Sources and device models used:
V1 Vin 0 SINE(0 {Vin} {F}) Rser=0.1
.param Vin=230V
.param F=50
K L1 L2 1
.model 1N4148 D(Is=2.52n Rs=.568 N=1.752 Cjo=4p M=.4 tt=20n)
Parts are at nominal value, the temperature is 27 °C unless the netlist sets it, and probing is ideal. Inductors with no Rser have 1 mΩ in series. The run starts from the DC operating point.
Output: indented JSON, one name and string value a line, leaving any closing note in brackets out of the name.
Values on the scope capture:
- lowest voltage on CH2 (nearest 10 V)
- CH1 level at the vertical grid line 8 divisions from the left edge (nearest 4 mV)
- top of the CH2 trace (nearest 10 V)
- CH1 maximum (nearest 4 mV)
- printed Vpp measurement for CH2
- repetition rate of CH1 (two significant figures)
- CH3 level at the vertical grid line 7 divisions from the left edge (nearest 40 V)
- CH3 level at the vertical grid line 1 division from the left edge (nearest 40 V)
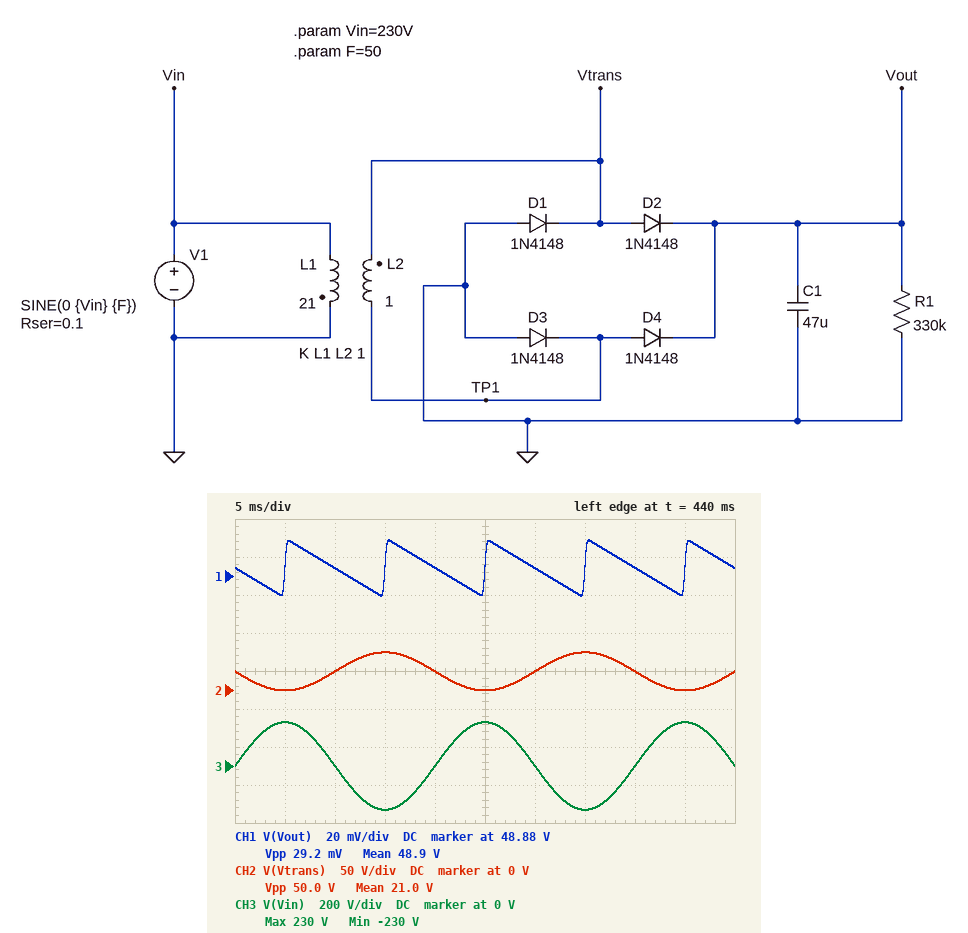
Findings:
{
  "lowest voltage on CH2": "0 V",
  "CH1 level at the vertical grid line 8 divisions from the left edge": "48.884 V",
  "top of the CH2 trace": "50 V",
  "CH1 maximum": "48.900 V",
  "printed Vpp measurement for CH2": "50.0 V",
  "repetition rate of CH1": "100 Hz",
  "CH3 level at the vertical grid line 7 divisions from the left edge": "-240 V",
  "CH3 level at the vertical grid line 1 division from the left edge": "240 V"
}
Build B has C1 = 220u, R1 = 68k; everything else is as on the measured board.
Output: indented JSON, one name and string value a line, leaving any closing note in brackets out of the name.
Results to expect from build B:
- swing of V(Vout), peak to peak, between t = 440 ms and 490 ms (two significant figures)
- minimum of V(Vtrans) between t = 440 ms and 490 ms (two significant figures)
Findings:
{
  "swing of V(Vout), peak to peak, between t = 440 ms and 490 ms": "30 mV",
  "minimum of V(Vtrans) between t = 440 ms and 490 ms": "-730 mV"
}
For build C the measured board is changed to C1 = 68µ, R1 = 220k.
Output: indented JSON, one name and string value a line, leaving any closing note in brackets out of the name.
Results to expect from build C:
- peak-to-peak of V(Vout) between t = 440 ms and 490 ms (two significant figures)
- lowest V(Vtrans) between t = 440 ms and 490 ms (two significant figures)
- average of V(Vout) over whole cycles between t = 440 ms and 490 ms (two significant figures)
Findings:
{
  "peak-to-peak of V(Vout) between t = 440 ms and 490 ms": "30 mV",
  "lowest V(Vtrans) between t = 440 ms and 490 ms": "-670 mV",
  "average of V(Vout) over whole cycles between t = 440 ms and 490 ms": "49 V"
}
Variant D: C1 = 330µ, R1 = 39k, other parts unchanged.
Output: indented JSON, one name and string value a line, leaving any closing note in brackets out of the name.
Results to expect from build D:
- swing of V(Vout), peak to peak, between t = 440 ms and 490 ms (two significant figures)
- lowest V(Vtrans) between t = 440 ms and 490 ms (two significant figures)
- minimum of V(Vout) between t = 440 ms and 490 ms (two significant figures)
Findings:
{
  "swing of V(Vout), peak to peak, between t = 440 ms and 490 ms": "35 mV",
  "lowest V(Vtrans) between t = 440 ms and 490 ms": "-760 mV",
  "minimum of V(Vout) between t = 440 ms and 490 ms": "49 V"
}
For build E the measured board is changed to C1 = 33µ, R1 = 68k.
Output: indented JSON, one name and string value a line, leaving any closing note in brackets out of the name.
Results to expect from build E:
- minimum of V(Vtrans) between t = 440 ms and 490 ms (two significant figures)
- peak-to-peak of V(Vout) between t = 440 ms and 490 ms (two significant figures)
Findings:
{
  "minimum of V(Vtrans) between t = 440 ms and 490 ms": "-730 mV",
  "peak-to-peak of V(Vout) between t = 440 ms and 490 ms": "200 mV"
}
